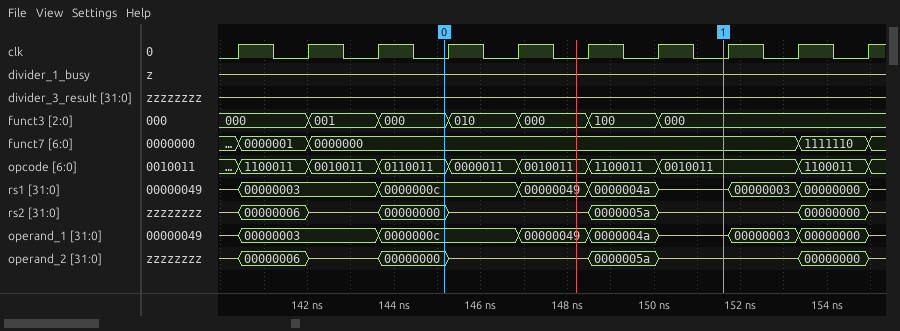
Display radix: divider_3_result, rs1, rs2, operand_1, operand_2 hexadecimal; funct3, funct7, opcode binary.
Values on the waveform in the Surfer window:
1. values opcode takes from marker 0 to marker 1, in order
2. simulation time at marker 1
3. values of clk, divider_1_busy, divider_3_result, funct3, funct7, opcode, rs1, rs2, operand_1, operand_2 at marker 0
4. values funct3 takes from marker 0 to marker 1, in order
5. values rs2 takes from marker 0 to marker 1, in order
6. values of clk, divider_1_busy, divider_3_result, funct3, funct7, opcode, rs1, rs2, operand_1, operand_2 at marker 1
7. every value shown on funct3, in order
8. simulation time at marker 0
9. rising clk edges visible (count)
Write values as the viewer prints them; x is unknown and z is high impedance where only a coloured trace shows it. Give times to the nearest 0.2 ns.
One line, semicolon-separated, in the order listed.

0110011, 0000011, 0010011, 1100011, 0010011; 151.6 ns; clk=0, divider_1_busy=z, divider_3_result=z, funct3=000, funct7=0000000, opcode=0110011, rs1=0000000c, rs2=00000000, operand_1=0000000c, operand_2=00000000; 000, 010, 000, 100, 000; 00000000, z, 0000005a, z; clk=0, divider_1_busy=z, divider_3_result=z, funct3=000, funct7=0000000, opcode=0010011, rs1=z, rs2=z, operand_1=z, operand_2=z; 000, 001, 000, 010, 000, 100, 000; 145.2 ns; 10
